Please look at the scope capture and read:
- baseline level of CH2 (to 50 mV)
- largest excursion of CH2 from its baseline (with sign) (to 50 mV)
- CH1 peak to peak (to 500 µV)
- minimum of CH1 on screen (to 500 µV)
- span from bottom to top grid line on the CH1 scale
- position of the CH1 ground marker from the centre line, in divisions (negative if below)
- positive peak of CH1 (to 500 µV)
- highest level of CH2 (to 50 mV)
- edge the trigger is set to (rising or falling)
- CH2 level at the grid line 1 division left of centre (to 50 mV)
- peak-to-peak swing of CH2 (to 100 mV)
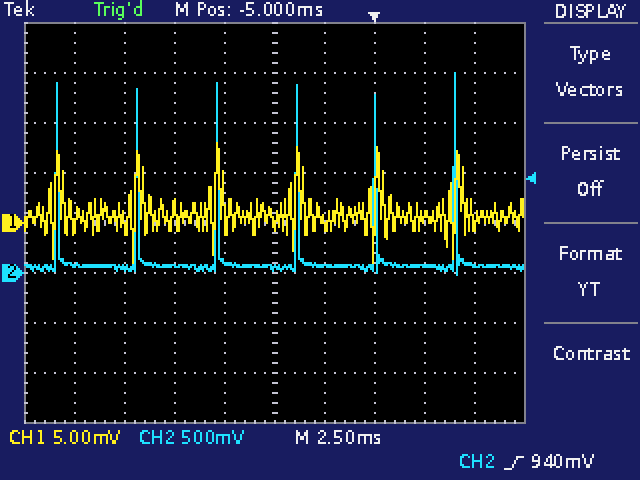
50 mV
+1.95 V
12.0 mV
-4.0 mV
40 mV
0.0 div
8.0 mV
2.00 V
rising
100 mV
2.00 V
